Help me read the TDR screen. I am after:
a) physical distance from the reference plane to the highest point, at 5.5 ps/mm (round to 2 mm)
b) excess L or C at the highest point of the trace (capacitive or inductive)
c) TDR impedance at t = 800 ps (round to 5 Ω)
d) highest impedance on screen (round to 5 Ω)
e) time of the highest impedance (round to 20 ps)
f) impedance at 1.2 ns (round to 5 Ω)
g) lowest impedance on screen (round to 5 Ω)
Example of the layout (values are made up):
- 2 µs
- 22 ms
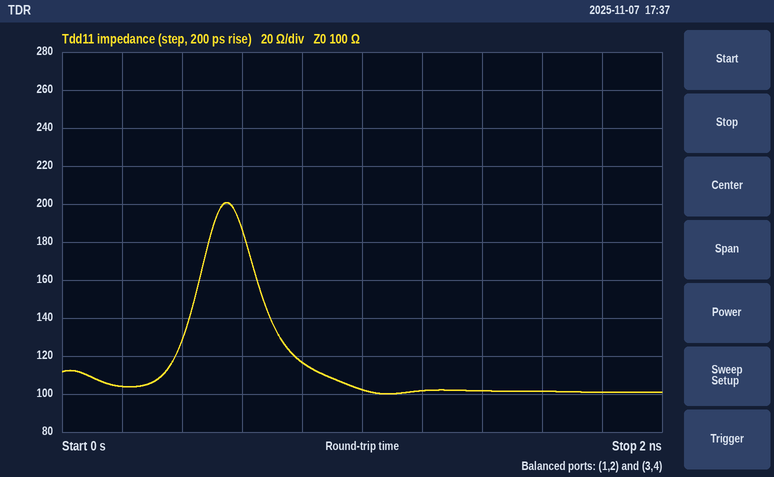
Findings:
- 50 mm
- inductive
- 115 Ω
- 200 Ω
- 540 ps
- 100 Ω
- 100 Ω
